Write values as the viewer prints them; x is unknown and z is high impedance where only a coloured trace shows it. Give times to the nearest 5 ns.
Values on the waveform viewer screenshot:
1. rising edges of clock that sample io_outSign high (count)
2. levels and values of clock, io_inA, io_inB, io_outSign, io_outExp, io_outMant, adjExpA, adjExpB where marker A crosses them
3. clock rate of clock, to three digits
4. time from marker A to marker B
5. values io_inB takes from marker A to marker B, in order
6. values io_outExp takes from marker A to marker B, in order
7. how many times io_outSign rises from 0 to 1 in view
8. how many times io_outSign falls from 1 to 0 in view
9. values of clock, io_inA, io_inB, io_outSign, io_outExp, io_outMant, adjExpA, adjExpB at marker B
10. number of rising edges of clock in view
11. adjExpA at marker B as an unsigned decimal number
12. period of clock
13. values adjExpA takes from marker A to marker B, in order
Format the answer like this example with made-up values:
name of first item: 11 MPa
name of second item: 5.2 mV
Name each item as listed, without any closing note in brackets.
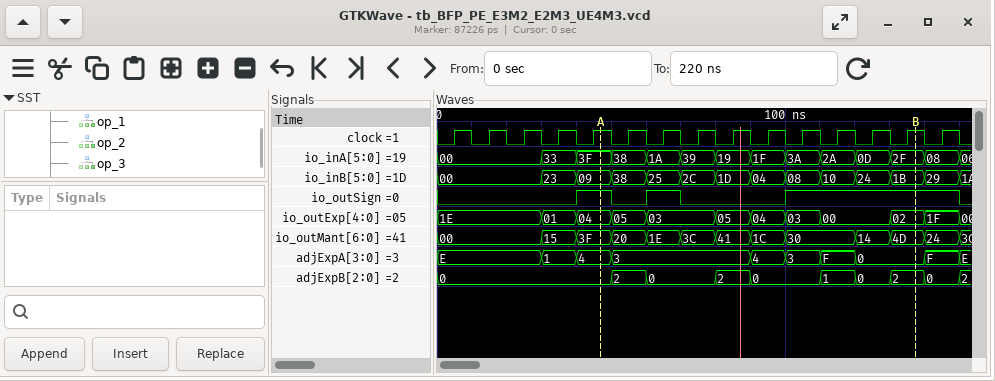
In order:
rising edges of clock that sample io_outSign high: 7
levels and values of clock, io_inA, io_inB, io_outSign, io_outExp, io_outMant, adjExpA, adjExpB where marker A crosses them: clock=1, io_inA=3F, io_inB=09, io_outSign=1, io_outExp=04, io_outMant=3F, adjExpA=4, adjExpB=0
clock rate of clock, to three digits: 100 MHz
time from marker A to marker B: 90 ns
values io_inB takes from marker A to marker B, in order: 09, 38, 25, 2C, 1D, 04, 08, 10, 24, 1B
values io_outExp takes from marker A to marker B, in order: 04, 05, 03, 05, 04, 03, 00, 02
how many times io_outSign rises from 0 to 1 in view: 3
how many times io_outSign falls from 1 to 0 in view: 3
values of clock, io_inA, io_inB, io_outSign, io_outExp, io_outMant, adjExpA, adjExpB at marker B: clock=1, io_inA=2F, io_inB=1B, io_outSign=1, io_outExp=02, io_outMant=4D, adjExpA=0, adjExpB=2
number of rising edges of clock in view: 15
adjExpA at marker B as an unsigned decimal number: 0
period of clock: 10 ns
values adjExpA takes from marker A to marker B, in order: 4, 3, 4, 3, F, 0
